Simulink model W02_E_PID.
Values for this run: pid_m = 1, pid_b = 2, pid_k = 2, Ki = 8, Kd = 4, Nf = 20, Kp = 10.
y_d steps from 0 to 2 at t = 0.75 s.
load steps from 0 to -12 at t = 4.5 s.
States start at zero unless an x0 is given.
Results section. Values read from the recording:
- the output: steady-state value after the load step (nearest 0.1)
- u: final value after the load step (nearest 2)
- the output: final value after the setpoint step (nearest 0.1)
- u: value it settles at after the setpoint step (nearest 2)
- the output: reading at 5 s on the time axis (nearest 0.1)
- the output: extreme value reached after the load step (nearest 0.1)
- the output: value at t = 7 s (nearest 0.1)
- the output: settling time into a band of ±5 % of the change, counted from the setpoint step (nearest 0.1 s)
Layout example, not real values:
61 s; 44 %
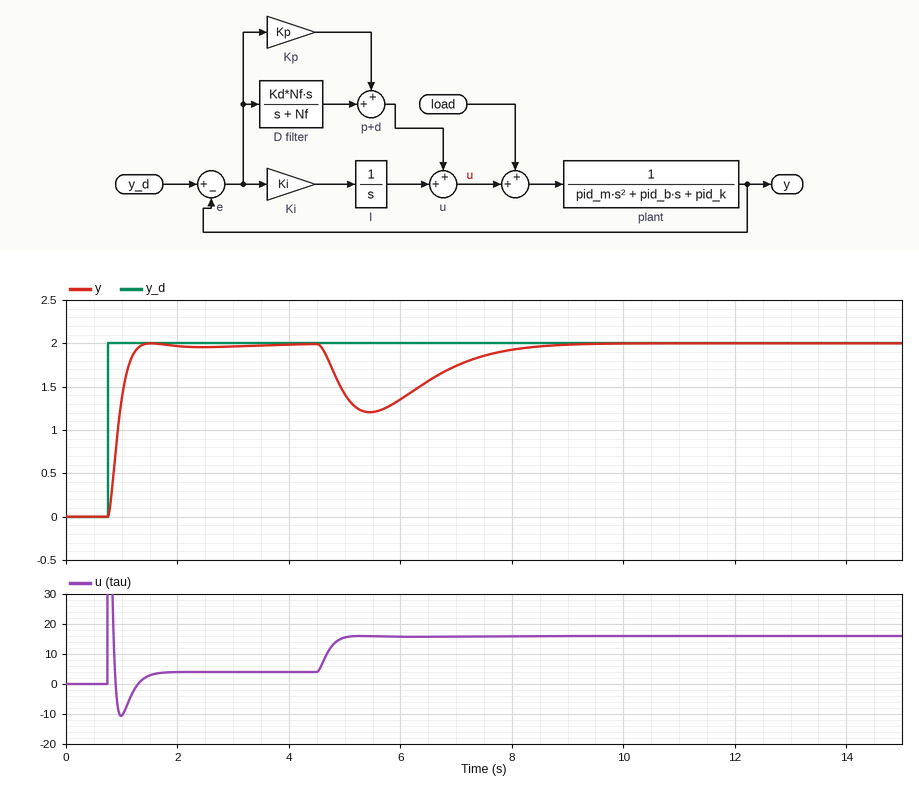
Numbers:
2.0; 16; 2.0; 4; 1.4; 1.2; 1.7; 0.5 s
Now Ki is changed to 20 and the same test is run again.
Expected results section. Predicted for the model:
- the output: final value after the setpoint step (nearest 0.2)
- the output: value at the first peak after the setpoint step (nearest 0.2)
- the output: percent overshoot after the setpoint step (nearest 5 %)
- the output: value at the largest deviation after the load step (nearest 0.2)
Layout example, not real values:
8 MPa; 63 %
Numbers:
2.0; 2.2; 15 %; 1.4
